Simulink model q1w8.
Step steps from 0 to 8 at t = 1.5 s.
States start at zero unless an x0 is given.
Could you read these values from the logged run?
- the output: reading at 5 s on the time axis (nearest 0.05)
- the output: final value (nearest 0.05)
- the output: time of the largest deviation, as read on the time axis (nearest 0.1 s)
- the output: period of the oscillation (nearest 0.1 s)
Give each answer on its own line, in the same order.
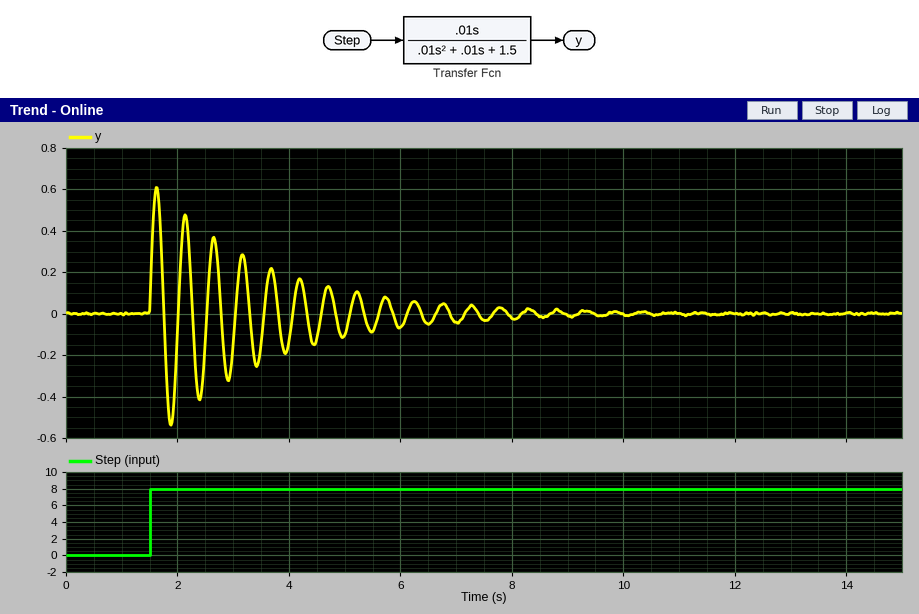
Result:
-0.10
0.00
1.6 s
0.5 s
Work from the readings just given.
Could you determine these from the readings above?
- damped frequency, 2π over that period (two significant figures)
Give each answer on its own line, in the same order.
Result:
13 rad/s
